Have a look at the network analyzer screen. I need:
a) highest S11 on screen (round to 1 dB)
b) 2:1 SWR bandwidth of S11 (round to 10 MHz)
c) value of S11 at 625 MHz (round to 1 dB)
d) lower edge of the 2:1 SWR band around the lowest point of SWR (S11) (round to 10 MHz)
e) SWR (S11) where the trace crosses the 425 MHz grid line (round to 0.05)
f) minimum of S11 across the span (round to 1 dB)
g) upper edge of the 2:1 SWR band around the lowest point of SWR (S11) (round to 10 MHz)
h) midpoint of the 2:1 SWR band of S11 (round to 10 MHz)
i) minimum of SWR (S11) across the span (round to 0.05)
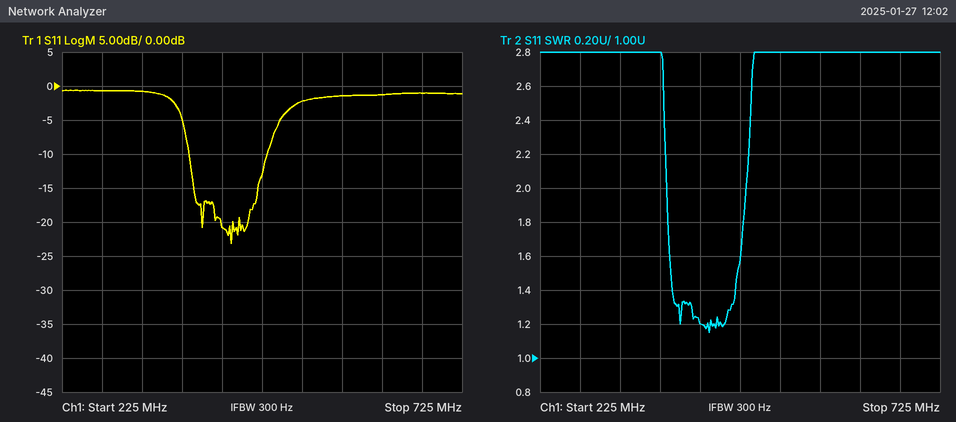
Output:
-1 dB
100 MHz
-1 dB
380 MHz
1.20
-23 dB
480 MHz
430 MHz
1.15
